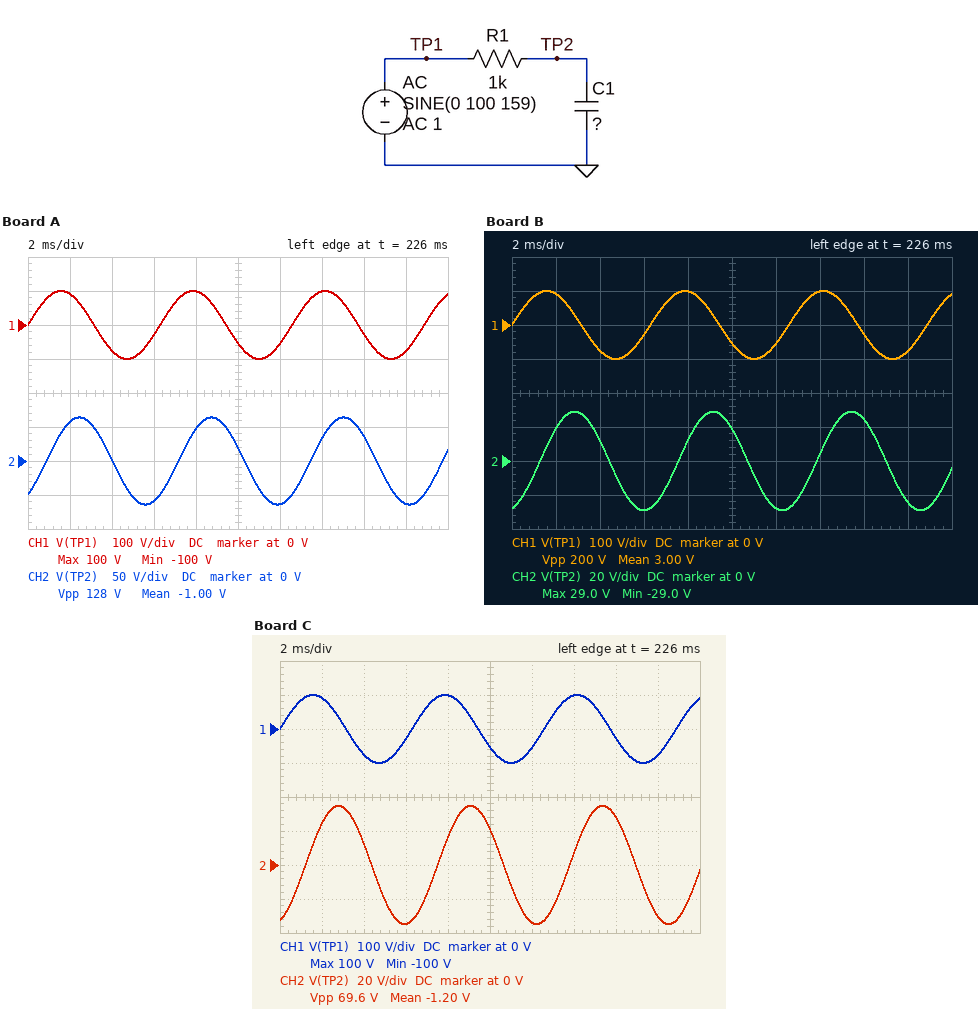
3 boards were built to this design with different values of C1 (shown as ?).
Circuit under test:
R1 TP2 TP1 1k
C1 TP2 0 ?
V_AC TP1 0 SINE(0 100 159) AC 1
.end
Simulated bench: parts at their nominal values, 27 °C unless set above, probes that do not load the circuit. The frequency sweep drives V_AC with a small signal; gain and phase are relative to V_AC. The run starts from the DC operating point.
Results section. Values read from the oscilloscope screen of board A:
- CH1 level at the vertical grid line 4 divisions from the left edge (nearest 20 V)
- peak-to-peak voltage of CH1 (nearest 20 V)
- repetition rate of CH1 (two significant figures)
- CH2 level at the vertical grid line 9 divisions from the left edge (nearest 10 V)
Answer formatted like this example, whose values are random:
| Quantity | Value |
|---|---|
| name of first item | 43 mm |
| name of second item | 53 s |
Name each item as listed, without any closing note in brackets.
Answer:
| Quantity | Value |
|---|---|
| CH1 level at the vertical grid line 4 divisions from the left edge | 100 V |
| peak-to-peak voltage of CH1 | 200 V |
| repetition rate of CH1 | 160 Hz |
| CH2 level at the vertical grid line 9 divisions from the left edge | -60 V |
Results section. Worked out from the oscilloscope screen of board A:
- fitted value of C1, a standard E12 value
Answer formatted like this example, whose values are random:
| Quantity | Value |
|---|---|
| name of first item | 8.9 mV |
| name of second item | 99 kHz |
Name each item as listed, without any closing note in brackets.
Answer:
| Quantity | Value |
|---|---|
| fitted value of C1, a standard E12 value | 1.2 µF |
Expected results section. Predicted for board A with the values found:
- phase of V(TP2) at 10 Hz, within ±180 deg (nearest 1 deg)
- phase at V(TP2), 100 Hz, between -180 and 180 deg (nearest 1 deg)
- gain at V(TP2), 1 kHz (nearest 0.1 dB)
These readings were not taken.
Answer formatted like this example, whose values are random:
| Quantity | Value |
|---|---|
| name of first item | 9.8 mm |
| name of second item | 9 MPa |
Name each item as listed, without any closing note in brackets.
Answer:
| Quantity | Value |
|---|---|
| phase of V(TP2) at 10 Hz, within ±180 deg | -4 deg |
| phase at V(TP2), 100 Hz, between -180 and 180 deg | -37 deg |
| gain at V(TP2), 1 kHz | -17.6 dB |
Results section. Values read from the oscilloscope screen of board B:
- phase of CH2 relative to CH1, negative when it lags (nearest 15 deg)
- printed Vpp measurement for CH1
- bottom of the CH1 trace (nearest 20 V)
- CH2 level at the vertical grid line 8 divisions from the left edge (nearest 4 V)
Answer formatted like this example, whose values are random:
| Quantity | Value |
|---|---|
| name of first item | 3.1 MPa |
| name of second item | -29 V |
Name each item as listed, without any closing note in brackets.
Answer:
| Quantity | Value |
|---|---|
| phase of CH2 relative to CH1, negative when it lags | -75 deg |
| printed Vpp measurement for CH1 | 200 V |
| bottom of the CH1 trace | -100 V |
| CH2 level at the vertical grid line 8 divisions from the left edge | 24 V |
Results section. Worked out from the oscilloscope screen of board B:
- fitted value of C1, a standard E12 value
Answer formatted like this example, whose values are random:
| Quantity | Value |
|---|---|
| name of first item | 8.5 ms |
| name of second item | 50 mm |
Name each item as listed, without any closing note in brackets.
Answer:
| Quantity | Value |
|---|---|
| fitted value of C1, a standard E12 value | 3.3 µF |
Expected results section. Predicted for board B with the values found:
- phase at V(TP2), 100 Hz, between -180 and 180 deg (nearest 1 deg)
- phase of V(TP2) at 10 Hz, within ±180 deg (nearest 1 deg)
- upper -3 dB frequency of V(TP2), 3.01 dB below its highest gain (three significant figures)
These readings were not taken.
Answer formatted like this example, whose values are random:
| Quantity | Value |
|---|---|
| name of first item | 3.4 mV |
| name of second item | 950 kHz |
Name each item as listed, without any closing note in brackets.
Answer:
| Quantity | Value |
|---|---|
| phase at V(TP2), 100 Hz, between -180 and 180 deg | -64 deg |
| phase of V(TP2) at 10 Hz, within ±180 deg | -12 deg |
| upper -3 dB frequency of V(TP2), 3.01 dB below its highest gain | 48.2 Hz |
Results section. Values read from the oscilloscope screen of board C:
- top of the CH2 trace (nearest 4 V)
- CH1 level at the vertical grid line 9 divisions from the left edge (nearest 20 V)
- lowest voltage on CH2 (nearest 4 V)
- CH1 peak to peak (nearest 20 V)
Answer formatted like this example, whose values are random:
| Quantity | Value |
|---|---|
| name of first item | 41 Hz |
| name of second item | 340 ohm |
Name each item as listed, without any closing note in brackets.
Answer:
| Quantity | Value |
|---|---|
| top of the CH2 trace | 36 V |
| CH1 level at the vertical grid line 9 divisions from the left edge | -80 V |
| lowest voltage on CH2 | -36 V |
| CH1 peak to peak | 200 V |
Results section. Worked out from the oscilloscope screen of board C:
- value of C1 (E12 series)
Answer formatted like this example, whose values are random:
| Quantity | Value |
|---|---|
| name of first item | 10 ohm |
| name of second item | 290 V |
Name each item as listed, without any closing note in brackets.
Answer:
| Quantity | Value |
|---|---|
| value of C1 | 2.7 µF |
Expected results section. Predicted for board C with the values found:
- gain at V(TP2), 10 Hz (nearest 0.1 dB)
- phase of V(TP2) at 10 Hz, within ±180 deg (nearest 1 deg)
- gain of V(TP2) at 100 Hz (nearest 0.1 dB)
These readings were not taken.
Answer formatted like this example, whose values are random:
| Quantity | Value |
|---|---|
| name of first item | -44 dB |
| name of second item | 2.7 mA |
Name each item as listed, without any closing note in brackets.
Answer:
| Quantity | Value |
|---|---|
| gain at V(TP2), 10 Hz | -0.1 dB |
| phase of V(TP2) at 10 Hz, within ±180 deg | -10 deg |
| gain of V(TP2) at 100 Hz | -5.9 dB |
